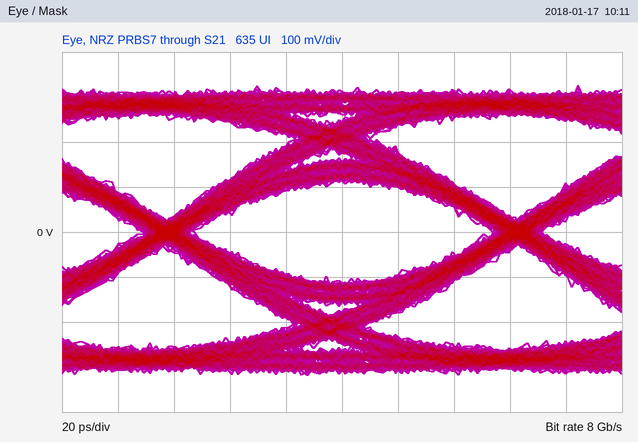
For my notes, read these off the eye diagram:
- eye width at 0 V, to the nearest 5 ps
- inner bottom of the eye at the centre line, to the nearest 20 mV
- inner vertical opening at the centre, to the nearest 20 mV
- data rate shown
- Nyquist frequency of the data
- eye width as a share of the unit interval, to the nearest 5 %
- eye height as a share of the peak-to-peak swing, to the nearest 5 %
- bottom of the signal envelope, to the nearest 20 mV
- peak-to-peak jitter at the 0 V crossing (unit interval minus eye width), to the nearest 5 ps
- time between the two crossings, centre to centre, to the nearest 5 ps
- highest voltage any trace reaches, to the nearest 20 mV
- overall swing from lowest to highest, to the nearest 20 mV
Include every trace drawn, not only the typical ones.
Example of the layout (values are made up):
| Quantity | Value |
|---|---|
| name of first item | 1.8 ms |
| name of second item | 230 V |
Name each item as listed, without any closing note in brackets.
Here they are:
| Quantity | Value |
|---|---|
| eye width at 0 V, to the nearest 5 ps | 105 ps |
| inner bottom of the eye at the centre line, to the nearest 20 mV | -120 mV |
| inner vertical opening at the centre, to the nearest 20 mV | 220 mV |
| data rate shown | 8 Gb/s |
| Nyquist frequency of the data | 4 GHz |
| eye width as a share of the unit interval, to the nearest 5 % | 85 % |
| eye height as a share of the peak-to-peak swing, to the nearest 5 % | 35 % |
| bottom of the signal envelope, to the nearest 20 mV | -320 mV |
| peak-to-peak jitter at the 0 V crossing (unit interval minus eye width), to the nearest 5 ps | 20 ps |
| time between the two crossings, centre to centre, to the nearest 5 ps | 125 ps |
| highest voltage any trace reaches, to the nearest 20 mV | 320 mV |
| overall swing from lowest to highest, to the nearest 20 mV | 640 mV |
